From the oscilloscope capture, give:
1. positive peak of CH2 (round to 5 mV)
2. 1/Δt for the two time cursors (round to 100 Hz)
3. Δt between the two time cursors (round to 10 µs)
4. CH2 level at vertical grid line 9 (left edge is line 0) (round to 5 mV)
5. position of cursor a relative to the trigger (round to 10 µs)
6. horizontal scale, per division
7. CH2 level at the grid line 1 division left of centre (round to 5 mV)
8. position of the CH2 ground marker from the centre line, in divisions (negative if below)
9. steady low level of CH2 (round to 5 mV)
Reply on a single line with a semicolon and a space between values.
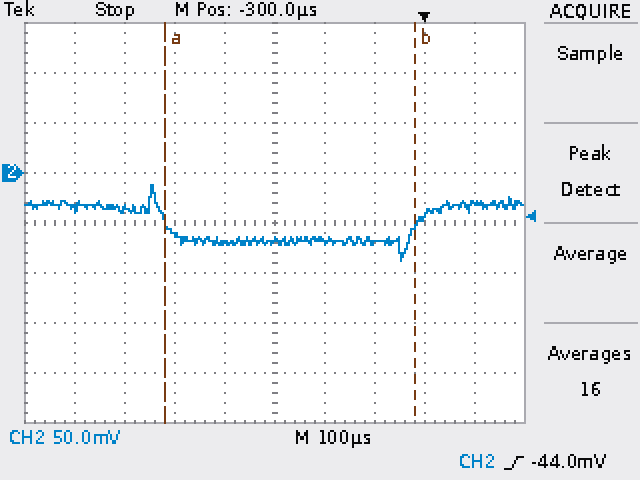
-10 mV; 2.0 kHz; 500 µs; -30 mV; -520 µs; 100 µs; -70 mV; +1.0 div; -70 mV
